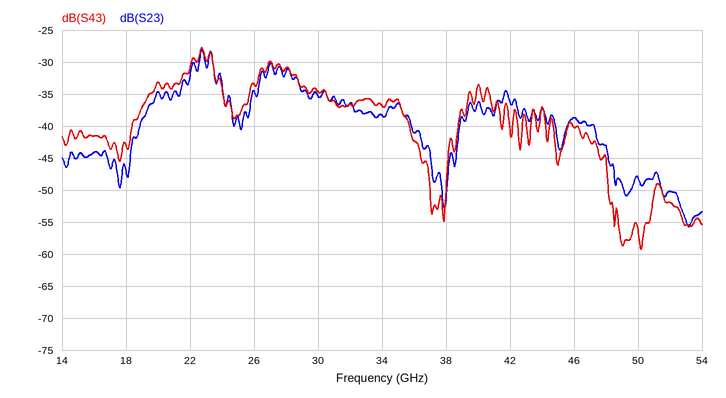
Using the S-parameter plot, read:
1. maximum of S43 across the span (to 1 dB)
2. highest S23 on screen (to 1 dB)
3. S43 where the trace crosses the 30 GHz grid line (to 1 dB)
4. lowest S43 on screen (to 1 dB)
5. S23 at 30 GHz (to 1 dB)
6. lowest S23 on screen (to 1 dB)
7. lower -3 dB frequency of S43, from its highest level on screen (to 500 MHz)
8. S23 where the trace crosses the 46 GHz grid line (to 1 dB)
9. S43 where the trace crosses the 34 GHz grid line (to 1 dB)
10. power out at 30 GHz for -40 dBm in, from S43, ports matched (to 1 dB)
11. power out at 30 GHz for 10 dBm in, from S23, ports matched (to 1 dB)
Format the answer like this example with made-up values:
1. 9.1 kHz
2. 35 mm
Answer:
1. -28 dB
2. -28 dB
3. -35 dB
4. -59 dB
5. -35 dB
6. -56 dB
7. 22.0 GHz
8. -39 dB
9. -37 dB
10. -75 dBm
11. -25 dBm
